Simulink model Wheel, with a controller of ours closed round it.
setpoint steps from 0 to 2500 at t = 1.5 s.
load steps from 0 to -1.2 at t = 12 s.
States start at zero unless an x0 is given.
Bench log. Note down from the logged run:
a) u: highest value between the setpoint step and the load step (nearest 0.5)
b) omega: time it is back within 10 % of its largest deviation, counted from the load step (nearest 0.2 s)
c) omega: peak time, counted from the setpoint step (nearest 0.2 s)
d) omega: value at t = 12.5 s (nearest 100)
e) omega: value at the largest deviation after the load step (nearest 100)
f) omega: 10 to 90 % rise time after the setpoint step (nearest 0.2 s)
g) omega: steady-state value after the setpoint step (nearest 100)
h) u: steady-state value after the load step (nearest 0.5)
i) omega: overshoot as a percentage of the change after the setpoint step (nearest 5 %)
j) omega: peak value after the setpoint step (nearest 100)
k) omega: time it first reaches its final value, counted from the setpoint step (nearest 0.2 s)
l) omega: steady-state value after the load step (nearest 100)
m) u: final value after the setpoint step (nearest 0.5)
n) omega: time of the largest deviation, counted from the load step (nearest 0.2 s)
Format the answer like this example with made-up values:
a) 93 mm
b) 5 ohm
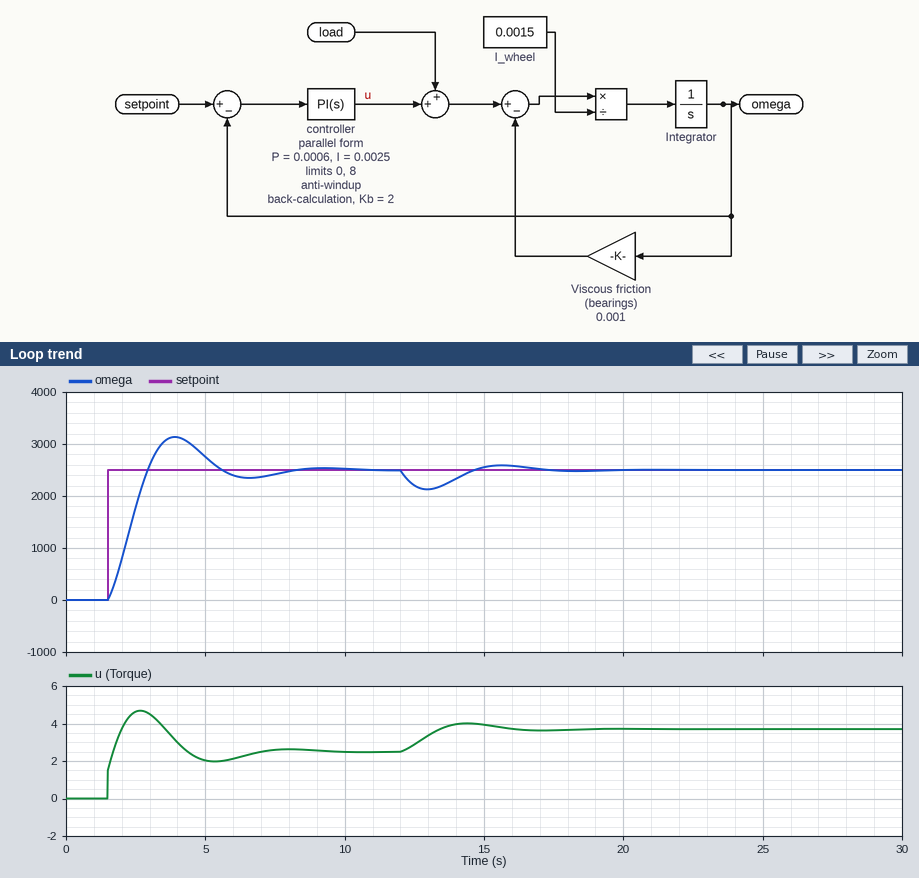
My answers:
a) 4.5
b) 4.8 s
c) 2.4 s
d) 2200
e) 2100
f) 1.0 s
g) 2500
h) 3.5
i) 25 %
j) 3100
k) 1.4 s
l) 2500
m) 2.5
n) 1.0 s
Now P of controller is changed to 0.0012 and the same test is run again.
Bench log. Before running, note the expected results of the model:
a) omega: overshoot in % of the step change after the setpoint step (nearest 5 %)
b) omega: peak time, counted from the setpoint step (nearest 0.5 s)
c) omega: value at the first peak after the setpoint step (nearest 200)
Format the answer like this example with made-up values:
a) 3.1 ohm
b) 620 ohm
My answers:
a) 15 %
b) 2.5 s
c) 2800
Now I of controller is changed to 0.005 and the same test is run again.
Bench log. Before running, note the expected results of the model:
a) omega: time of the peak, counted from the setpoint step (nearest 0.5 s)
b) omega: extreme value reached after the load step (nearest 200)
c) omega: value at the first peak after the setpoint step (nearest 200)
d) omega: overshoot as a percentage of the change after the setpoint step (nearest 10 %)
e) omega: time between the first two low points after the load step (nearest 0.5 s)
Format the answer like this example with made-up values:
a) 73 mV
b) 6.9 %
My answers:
a) 1.5 s
b) 2200
c) 3400
d) 40 %
e) 3.5 s
